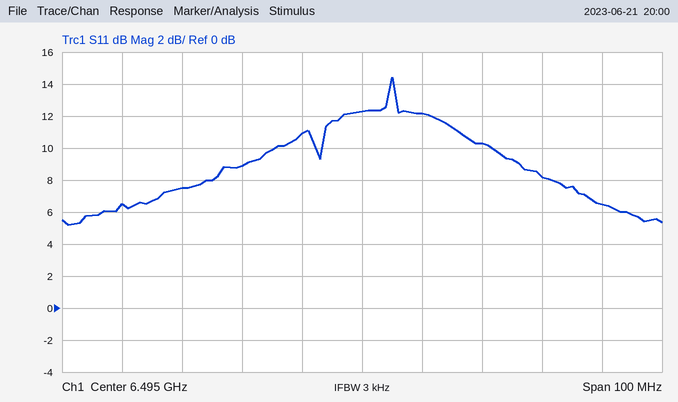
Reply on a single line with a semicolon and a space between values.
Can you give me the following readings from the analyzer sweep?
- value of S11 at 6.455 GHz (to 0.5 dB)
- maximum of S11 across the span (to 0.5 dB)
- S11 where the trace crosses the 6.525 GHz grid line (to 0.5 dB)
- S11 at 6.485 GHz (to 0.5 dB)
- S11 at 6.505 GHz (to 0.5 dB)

6.5 dB; 14.5 dB; 8.0 dB; 11.0 dB; 12.0 dB
